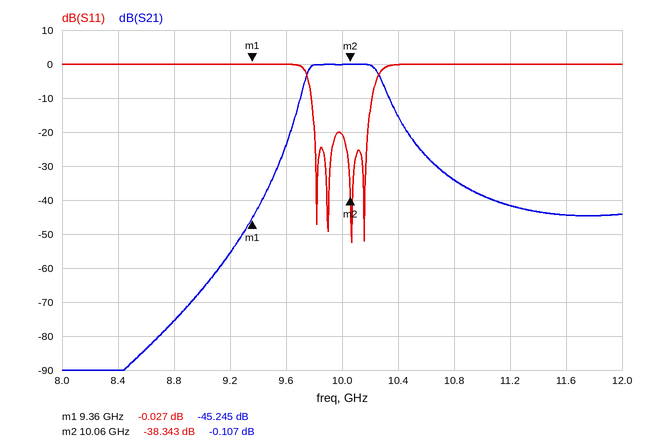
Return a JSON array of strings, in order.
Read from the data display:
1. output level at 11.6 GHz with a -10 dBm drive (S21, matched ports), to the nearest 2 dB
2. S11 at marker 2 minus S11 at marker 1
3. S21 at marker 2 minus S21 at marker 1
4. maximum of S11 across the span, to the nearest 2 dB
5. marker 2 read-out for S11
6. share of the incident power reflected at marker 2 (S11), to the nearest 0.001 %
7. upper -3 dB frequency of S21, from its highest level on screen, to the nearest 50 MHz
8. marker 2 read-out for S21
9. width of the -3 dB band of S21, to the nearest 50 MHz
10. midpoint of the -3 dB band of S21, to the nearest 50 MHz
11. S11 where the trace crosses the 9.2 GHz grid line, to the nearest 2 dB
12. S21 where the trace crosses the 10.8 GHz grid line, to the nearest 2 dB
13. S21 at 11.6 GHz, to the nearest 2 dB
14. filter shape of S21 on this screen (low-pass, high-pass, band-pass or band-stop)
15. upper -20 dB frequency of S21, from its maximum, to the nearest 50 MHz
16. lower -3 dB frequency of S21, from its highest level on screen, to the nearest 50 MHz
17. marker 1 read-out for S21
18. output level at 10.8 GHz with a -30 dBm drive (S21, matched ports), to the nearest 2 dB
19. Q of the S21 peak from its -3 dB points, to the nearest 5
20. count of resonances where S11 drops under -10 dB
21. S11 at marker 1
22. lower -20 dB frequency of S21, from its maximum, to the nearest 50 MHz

["-54 dBm", "-38.316 dB", "45.138 dB", "0 dB", "-38.343 dB", "0.015 %", "10.25 GHz", "-0.107 dB", "500 MHz", "10.00 GHz", "0 dB", "-34 dB", "-44 dB", "band-pass", "10.45 GHz", "9.75 GHz", "-45.245 dB", "-64 dBm", "20", "4", "-0.027 dB", "9.65 GHz"]
